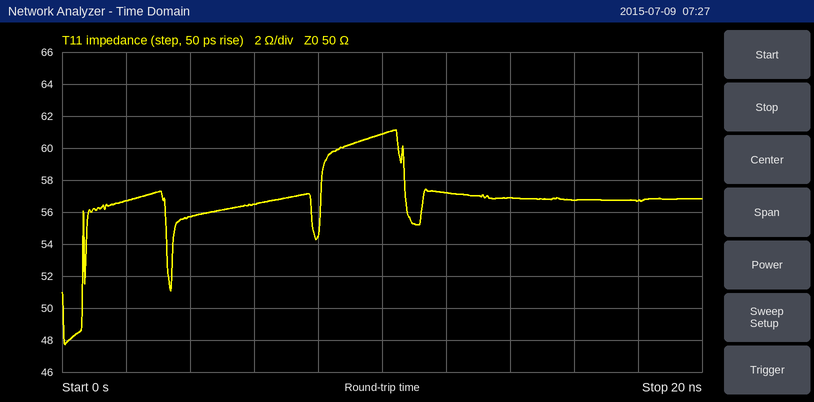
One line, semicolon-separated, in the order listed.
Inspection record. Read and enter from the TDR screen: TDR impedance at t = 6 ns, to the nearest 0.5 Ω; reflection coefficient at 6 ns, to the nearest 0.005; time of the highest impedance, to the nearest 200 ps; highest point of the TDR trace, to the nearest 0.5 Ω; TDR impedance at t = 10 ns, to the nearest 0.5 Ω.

56.5 Ω; +0.060; 10.4 ns; 61.0 Ω; 61.0 Ω
